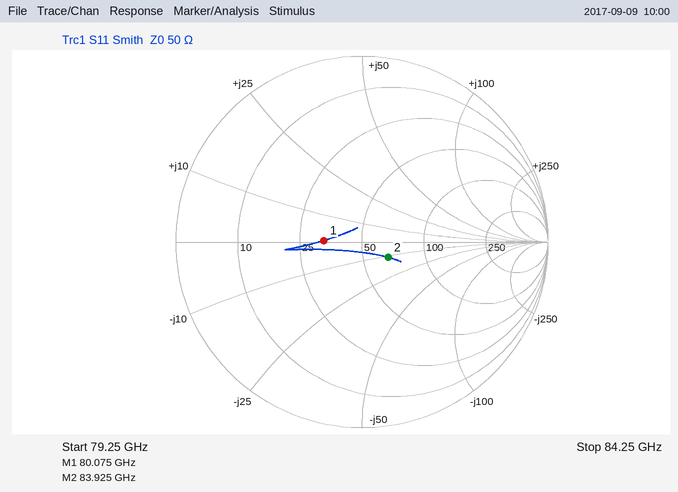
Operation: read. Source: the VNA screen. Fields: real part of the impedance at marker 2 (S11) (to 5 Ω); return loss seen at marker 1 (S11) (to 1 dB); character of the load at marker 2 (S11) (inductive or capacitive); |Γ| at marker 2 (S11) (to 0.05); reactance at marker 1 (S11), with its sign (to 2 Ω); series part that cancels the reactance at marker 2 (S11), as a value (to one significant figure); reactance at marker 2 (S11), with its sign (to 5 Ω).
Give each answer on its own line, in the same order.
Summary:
65 Ω
14 dB
capacitive
0.15
0 Ω
20 pH
-10 Ω
